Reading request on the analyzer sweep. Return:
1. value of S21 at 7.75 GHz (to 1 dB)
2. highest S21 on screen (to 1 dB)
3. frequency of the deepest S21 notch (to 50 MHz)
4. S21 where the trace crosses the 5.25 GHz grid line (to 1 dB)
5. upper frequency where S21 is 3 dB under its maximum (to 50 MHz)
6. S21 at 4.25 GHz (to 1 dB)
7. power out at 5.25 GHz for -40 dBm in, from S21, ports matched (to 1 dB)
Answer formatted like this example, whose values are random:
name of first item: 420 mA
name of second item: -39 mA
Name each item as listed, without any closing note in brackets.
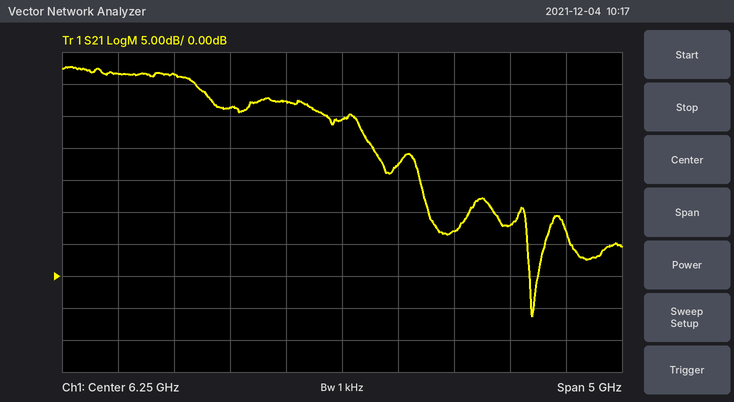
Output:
value of S21 at 7.75 GHz: 8 dB
highest S21 on screen: 33 dB
frequency of the deepest S21 notch: 7.95 GHz
S21 where the trace crosses the 5.25 GHz grid line: 26 dB
upper frequency where S21 is 3 dB under its maximum: 4.95 GHz
S21 at 4.25 GHz: 32 dB
power out at 5.25 GHz for -40 dBm in, from S21, ports matched: -14 dBm
